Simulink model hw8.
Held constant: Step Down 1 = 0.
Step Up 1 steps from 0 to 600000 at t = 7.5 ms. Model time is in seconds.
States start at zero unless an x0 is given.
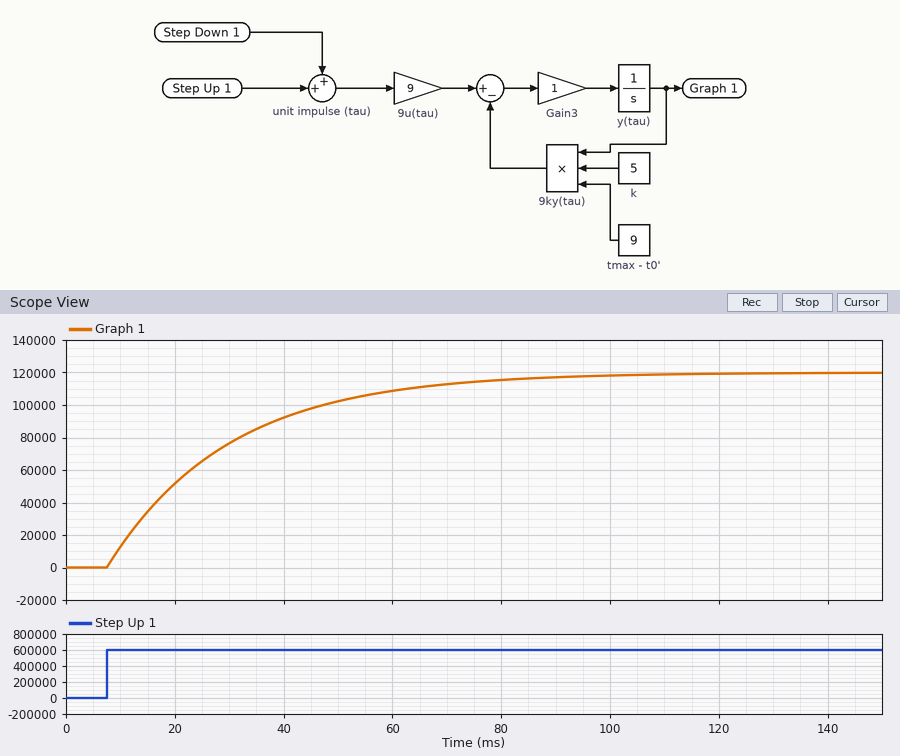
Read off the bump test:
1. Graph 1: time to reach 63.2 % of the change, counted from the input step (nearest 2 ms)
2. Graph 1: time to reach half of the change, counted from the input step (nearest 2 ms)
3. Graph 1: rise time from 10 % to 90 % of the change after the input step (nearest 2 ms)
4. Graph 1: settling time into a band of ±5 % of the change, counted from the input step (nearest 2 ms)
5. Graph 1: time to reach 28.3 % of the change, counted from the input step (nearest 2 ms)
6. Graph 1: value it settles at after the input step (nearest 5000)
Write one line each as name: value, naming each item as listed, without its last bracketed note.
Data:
Graph 1: time to reach 63.2 % of the change, counted from the input step: 22 ms
Graph 1: time to reach half of the change, counted from the input step: 16 ms
Graph 1: rise time from 10 % to 90 % of the change after the input step: 48 ms
Graph 1: settling time into a band of ±5 % of the change, counted from the input step: 66 ms
Graph 1: time to reach 28.3 % of the change, counted from the input step: 8 ms
Graph 1: value it settles at after the input step: 120000
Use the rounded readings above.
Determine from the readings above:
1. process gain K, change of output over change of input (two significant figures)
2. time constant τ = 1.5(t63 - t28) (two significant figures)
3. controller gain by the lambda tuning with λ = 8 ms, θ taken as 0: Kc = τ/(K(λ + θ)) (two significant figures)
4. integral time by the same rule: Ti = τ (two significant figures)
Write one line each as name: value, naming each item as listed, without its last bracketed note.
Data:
process gain K, change of output over change of input: 0.20
time constant τ = 1.5(t63 - t28): 21 ms
controller gain by the lambda tuning with λ = 8 ms, θ taken as 0: Kc = τ/(K(λ + θ)): 13
integral time by the same rule: Ti = τ: 21 ms
